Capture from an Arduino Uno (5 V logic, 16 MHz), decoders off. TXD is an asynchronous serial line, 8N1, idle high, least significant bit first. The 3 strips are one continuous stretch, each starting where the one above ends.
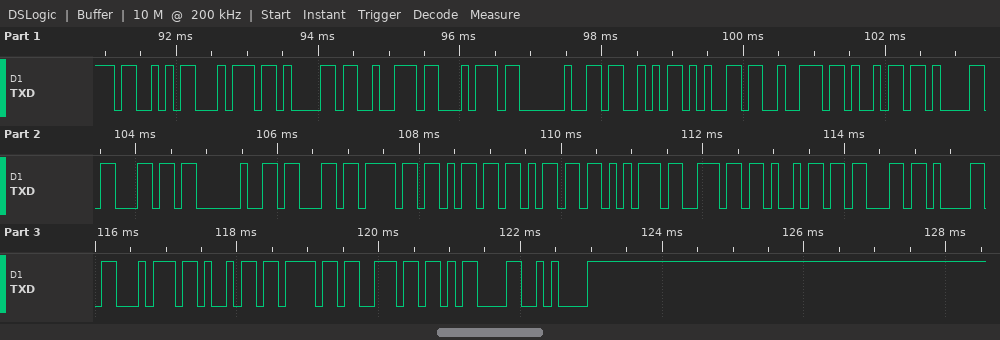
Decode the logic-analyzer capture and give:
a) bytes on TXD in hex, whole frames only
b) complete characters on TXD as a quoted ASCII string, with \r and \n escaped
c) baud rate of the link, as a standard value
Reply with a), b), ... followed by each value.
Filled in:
a) 53 74 61 72 74 20 53 65 72 69 61 6C 20 63 6F 6D 6D 75 6E 69 63 61 74 69 6F 6E 0D 0A
b) "Start Serial communication\r\n"
c) 9600 baud
